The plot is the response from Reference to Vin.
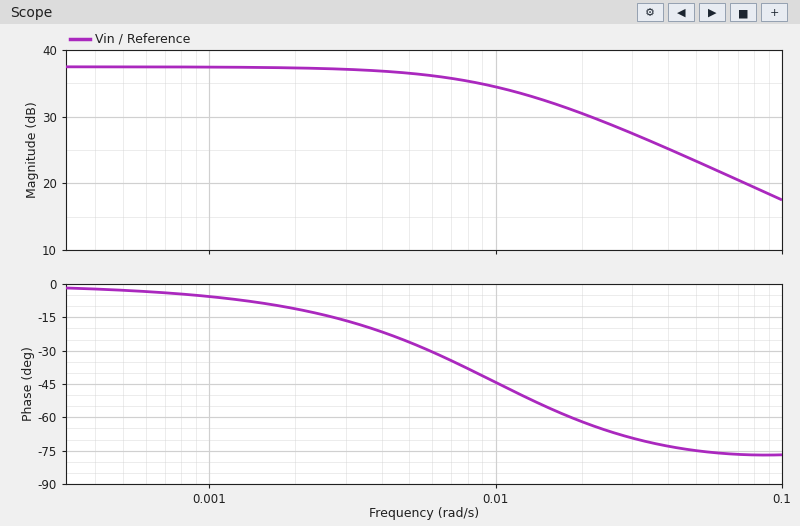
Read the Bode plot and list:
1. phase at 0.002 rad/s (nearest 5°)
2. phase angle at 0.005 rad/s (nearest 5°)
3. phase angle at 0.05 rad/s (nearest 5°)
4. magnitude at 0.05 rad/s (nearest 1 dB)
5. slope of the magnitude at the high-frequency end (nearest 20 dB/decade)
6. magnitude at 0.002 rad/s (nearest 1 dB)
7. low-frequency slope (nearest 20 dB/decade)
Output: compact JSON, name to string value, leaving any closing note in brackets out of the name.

{"phase at 0.002 rad/s": "-10°", "phase angle at 0.005 rad/s": "-25°", "phase angle at 0.05 rad/s": "-75°", "magnitude at 0.05 rad/s": "23 dB", "slope of the magnitude at the high-frequency end": "-20 dB/decade", "magnitude at 0.002 rad/s": "37 dB", "low-frequency slope": "0 dB/decade"}
